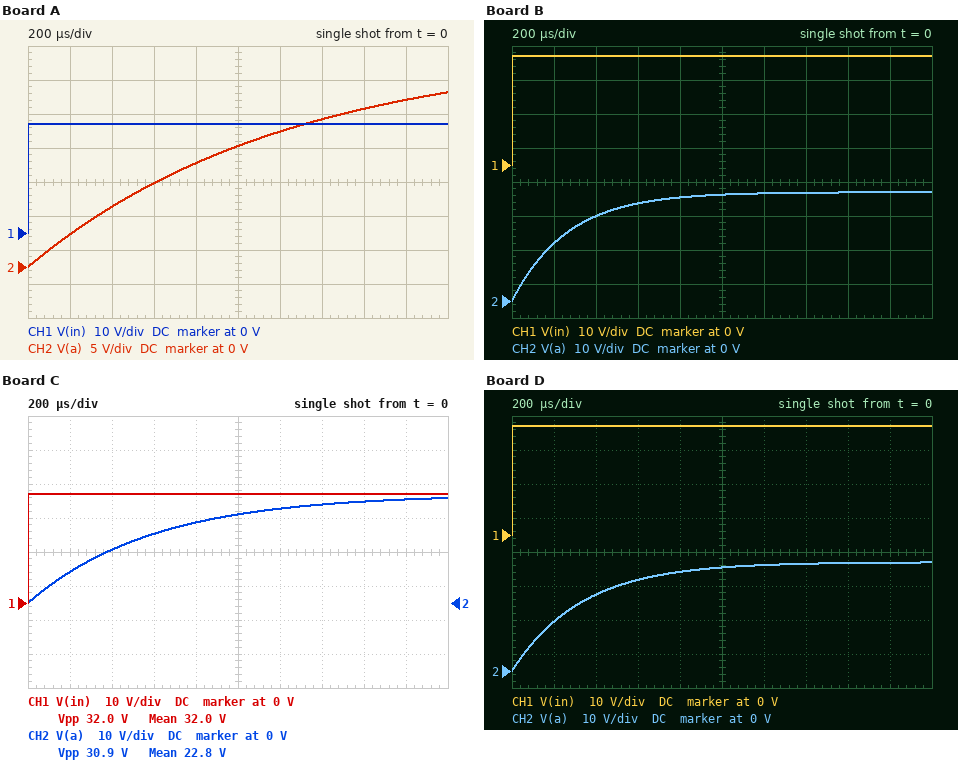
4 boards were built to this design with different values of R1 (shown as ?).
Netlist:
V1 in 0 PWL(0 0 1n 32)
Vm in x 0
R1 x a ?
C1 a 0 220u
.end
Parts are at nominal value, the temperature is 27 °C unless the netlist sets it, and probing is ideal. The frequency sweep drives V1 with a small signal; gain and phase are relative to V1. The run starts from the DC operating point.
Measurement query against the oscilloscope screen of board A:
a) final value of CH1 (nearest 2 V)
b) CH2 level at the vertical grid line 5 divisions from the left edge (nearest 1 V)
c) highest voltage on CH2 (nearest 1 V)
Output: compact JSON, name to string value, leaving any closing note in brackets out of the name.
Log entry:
{"final value of CH1": "32 V", "CH2 level at the vertical grid line 5 divisions from the left edge": "18 V", "highest voltage on CH2": "26 V"}
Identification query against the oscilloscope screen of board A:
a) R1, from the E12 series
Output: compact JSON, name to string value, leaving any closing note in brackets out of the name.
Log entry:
{"R1, from the E12 series": "5.6 Ω"}
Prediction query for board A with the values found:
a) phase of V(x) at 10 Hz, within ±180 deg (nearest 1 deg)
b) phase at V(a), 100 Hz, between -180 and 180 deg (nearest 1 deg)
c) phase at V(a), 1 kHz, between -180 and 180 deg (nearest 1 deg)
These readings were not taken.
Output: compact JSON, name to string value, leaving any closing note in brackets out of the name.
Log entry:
{"phase of V(x) at 10 Hz, within ±180 deg": "0 deg", "phase at V(a), 100 Hz, between -180 and 180 deg": "-38 deg", "phase at V(a), 1 kHz, between -180 and 180 deg": "-83 deg"}
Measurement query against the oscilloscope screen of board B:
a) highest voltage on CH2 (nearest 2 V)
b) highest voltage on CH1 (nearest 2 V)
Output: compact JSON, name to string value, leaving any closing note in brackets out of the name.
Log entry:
{"highest voltage on CH2": "32 V", "highest voltage on CH1": "32 V"}
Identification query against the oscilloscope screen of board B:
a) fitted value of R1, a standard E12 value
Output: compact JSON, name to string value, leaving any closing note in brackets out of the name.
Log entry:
{"fitted value of R1, a standard E12 value": "1.2 Ω"}
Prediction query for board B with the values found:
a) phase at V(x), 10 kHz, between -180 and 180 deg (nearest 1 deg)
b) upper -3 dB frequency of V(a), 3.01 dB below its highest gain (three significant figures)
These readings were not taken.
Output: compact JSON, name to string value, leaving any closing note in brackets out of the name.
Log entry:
{"phase at V(x), 10 kHz, between -180 and 180 deg": "0 deg", "upper -3 dB frequency of V(a), 3.01 dB below its highest gain": "603 Hz"}
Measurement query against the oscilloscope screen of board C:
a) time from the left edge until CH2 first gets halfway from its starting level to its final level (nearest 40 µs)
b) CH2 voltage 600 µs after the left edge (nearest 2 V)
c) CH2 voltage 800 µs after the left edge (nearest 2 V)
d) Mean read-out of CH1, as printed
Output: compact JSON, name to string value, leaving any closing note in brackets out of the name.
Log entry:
{"time from the left edge until CH2 first gets halfway from its starting level to its final level": "400 µs", "CH2 voltage 600 µs after the left edge": "20 V", "CH2 voltage 800 µs after the left edge": "24 V", "Mean read-out of CH1, as printed": "32.0 V"}
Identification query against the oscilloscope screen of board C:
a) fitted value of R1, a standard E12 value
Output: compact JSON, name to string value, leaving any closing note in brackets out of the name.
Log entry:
{"fitted value of R1, a standard E12 value": "2.7 Ω"}
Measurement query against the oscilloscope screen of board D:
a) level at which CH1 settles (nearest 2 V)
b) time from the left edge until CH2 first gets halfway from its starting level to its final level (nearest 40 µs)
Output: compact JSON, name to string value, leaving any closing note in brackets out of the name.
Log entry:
{"level at which CH1 settles": "32 V", "time from the left edge until CH2 first gets halfway from its starting level to its final level": "240 µs"}
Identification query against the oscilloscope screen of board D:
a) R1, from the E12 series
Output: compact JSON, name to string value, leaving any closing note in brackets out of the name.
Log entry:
{"R1, from the E12 series": "1.5 Ω"}
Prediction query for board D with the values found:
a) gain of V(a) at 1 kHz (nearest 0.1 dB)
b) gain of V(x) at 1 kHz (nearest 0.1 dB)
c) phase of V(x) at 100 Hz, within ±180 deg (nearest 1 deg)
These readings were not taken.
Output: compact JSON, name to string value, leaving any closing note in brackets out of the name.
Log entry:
{"gain of V(a) at 1 kHz": "-7.2 dB", "gain of V(x) at 1 kHz": "0 dB", "phase of V(x) at 100 Hz, within ±180 deg": "0 deg"}
